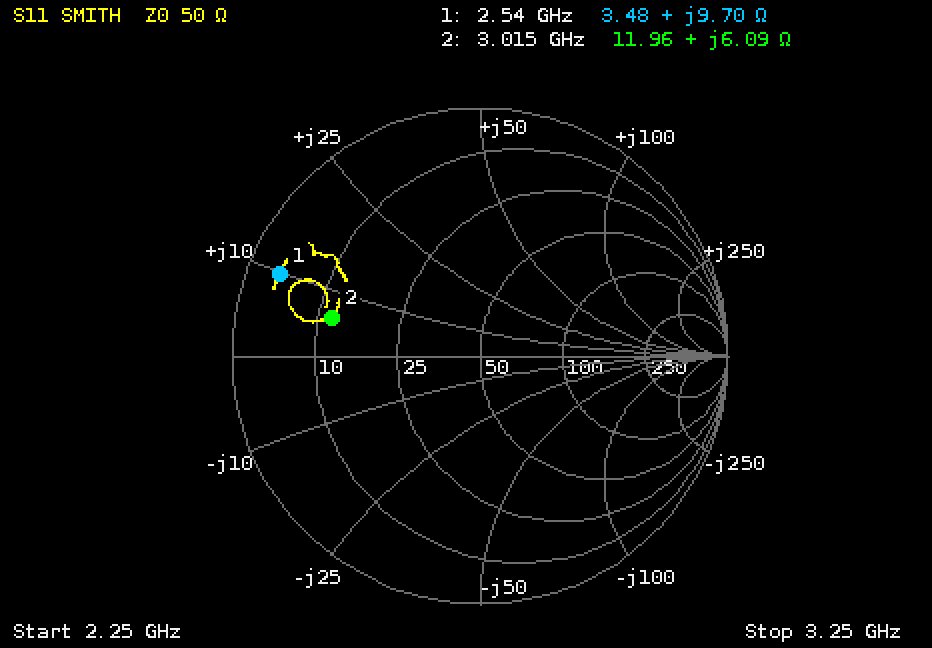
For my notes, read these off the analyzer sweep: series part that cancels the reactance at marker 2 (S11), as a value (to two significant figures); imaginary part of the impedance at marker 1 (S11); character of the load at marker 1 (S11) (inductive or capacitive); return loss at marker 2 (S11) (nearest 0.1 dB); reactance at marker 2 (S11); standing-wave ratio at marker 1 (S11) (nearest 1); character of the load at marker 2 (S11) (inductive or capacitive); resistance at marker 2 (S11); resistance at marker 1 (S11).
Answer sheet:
8.7 pF
+9.70 Ω
inductive
4.2 dB
+6.09 Ω
15
inductive
11.96 Ω
3.48 Ω
